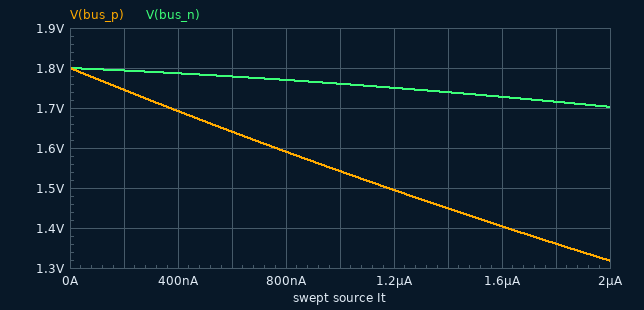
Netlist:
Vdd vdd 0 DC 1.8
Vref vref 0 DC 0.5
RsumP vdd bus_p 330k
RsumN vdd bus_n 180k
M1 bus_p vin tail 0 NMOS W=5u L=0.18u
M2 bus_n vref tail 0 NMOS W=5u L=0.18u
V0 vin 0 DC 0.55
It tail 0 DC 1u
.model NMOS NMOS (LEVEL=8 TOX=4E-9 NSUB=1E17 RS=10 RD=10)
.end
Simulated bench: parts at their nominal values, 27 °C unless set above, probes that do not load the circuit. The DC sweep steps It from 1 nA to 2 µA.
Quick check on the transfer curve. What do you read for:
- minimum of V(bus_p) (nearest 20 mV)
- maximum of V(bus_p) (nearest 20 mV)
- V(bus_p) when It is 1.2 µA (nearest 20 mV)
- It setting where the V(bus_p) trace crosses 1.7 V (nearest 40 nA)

1.32 V
1.80 V
1.50 V
360 nA
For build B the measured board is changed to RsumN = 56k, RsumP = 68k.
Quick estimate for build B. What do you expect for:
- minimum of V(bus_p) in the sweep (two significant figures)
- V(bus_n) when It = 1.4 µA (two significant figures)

1.7 V
1.8 V
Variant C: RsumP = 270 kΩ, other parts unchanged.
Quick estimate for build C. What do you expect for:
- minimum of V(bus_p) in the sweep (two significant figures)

1.4 V
